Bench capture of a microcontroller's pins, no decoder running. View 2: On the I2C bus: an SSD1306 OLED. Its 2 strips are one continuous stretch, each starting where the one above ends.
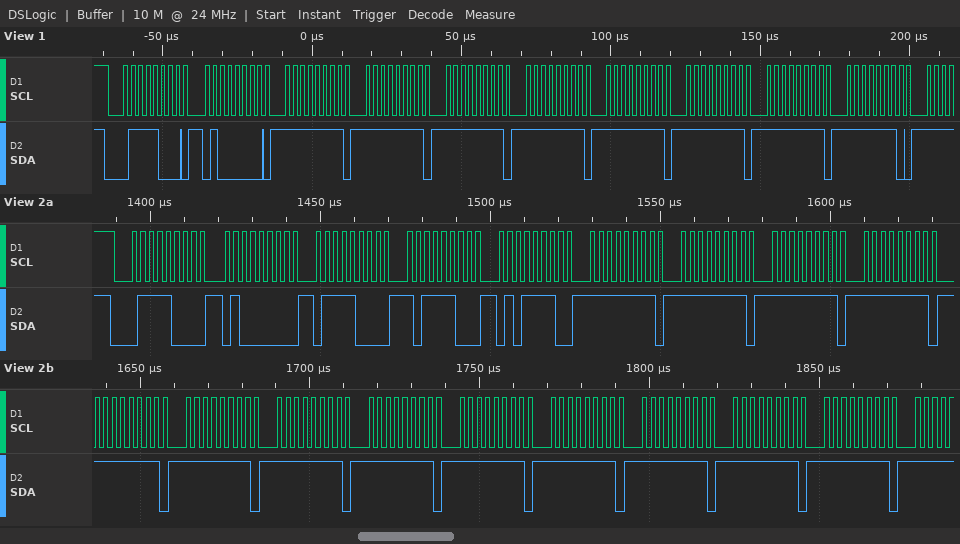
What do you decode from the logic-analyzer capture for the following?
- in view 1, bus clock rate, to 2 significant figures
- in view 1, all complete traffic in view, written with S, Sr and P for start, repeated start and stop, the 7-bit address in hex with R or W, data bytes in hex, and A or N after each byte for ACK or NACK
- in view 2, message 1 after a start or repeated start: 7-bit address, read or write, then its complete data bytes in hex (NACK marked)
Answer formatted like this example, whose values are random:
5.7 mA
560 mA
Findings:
400 kHz
S 3CW A 40 A FF A FF A FF A FF A FF A FF A FF A FE A
0x3C write: 40 78 BC 5E FF FF FF FF FF FF FF FF FF FF FF FF FF
